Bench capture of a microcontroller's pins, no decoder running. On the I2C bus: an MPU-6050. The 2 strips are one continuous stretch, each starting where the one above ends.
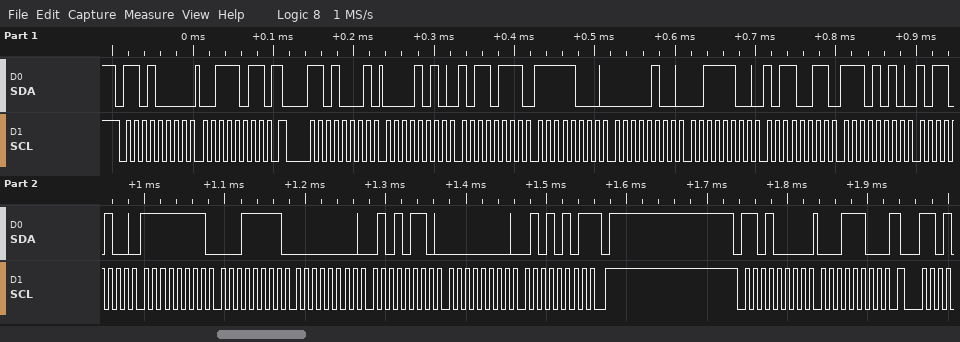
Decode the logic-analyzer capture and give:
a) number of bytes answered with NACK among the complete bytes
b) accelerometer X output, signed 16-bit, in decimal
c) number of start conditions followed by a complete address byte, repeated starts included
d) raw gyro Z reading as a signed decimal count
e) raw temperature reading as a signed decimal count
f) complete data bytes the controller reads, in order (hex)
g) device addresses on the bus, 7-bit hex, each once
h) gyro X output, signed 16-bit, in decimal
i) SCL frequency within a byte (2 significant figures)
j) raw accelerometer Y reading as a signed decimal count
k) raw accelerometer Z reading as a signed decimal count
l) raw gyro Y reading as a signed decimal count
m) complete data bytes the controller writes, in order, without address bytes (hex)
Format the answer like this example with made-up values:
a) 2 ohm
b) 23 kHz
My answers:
a) 1
b) 2743
c) 3
d) 85
e) -5452
f) 0A B7 F8 04 3C B3 EA B4 FF 1F 00 56 00 55
g) 0x68
h) -225
i) 100 kHz
j) -2044
k) 15539
l) 86
m) 3B 1C
